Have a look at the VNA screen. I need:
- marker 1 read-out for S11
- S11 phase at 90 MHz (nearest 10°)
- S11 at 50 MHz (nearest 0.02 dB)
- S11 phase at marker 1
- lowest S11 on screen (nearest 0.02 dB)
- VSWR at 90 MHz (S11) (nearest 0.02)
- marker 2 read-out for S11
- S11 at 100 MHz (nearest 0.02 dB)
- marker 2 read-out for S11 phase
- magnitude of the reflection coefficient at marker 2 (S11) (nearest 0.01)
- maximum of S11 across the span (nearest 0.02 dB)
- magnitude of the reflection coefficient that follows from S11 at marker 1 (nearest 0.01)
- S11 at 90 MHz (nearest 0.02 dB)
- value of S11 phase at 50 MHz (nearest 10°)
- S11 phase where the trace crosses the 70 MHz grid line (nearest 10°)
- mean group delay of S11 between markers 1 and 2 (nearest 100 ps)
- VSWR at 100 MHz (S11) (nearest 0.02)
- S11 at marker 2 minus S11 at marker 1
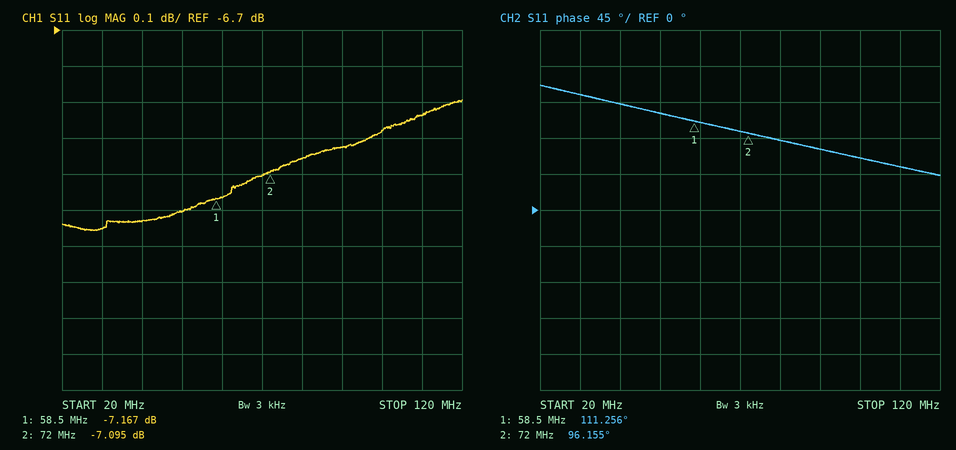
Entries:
-7.167 dB
80°
-7.20 dB
111.256°
-7.26 dB
2.60
-7.095 dB
-6.98 dB
96.155°
0.44
-6.90 dB
0.44
-7.02 dB
120°
100°
3.1 ns
2.62
0.072 dB
